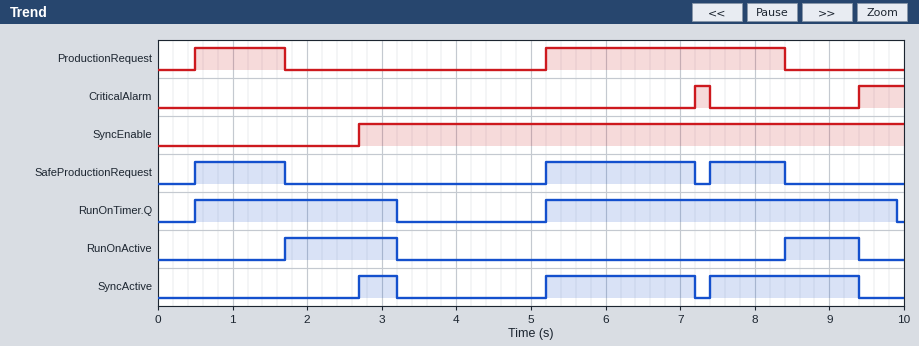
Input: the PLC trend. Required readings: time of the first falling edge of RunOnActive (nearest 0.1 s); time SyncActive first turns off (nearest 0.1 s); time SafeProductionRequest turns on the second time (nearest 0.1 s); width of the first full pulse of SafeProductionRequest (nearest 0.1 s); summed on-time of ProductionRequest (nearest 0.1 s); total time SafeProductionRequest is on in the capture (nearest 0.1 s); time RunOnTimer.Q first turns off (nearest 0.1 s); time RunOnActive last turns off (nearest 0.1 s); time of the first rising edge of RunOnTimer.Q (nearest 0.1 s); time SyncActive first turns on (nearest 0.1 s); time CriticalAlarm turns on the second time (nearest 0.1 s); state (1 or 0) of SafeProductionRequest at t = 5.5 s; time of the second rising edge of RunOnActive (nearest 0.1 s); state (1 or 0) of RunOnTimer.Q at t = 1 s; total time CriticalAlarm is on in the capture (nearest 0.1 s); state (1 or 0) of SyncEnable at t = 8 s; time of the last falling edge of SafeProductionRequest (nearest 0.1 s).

3.2 s
3.2 s
5.2 s
1.2 s
4.4 s
4.2 s
3.2 s
9.4 s
0.5 s
2.7 s
9.4 s
1
8.4 s
1
0.8 s
1
8.4 s
